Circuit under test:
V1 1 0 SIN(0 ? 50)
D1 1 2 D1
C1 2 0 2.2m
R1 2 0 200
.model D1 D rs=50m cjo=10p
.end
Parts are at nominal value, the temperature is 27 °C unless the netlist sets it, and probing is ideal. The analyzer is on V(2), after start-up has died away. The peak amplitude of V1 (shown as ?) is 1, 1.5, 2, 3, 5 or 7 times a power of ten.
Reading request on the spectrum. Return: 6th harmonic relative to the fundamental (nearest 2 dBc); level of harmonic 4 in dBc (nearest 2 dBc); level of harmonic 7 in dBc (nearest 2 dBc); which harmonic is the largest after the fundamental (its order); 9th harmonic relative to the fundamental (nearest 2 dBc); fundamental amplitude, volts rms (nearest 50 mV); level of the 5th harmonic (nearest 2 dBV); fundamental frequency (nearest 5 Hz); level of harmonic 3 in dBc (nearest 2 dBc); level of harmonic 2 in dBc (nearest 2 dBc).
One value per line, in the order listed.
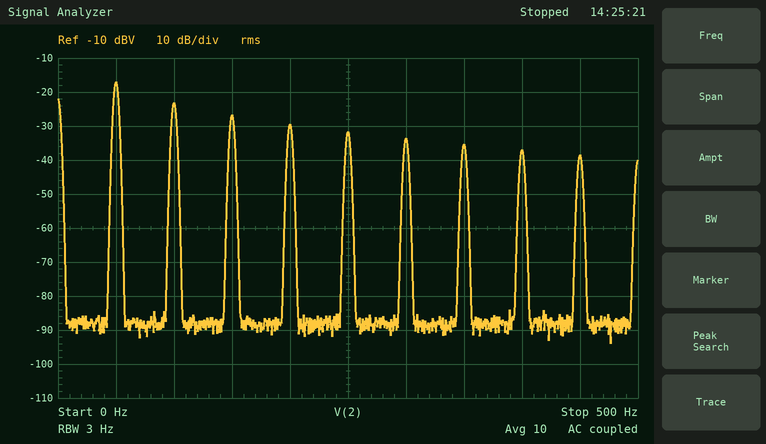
-16 dBc
-12 dBc
-18 dBc
2
-22 dBc
150 mV
-32 dBV
50 Hz
-10 dBc
-6 dBc
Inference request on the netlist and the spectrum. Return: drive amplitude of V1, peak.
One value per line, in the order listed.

15 V
